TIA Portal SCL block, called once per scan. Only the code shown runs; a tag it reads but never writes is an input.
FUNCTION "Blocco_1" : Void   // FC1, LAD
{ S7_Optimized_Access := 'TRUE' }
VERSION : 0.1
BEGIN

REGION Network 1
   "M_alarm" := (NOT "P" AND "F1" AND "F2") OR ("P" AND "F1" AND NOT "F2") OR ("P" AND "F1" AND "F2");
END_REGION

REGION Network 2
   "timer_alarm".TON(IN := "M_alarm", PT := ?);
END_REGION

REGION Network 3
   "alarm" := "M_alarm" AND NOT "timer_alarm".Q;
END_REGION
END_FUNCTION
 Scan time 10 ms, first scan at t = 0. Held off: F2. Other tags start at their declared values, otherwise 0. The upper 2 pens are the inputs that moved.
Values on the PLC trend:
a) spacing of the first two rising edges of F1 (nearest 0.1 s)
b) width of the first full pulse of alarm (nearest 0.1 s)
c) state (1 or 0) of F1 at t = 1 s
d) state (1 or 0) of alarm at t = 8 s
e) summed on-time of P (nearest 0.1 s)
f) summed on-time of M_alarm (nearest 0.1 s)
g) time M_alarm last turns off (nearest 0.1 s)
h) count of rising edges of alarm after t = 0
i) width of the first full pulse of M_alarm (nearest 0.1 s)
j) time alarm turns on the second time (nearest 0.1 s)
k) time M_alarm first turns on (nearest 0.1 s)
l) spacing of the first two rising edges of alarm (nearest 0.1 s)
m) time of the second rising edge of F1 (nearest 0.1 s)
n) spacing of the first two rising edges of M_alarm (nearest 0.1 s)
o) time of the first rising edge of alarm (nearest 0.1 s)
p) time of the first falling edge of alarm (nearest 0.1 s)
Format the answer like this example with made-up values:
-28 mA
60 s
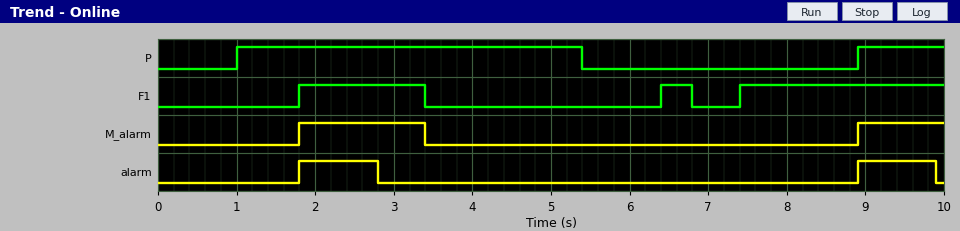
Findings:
4.6 s
1.0 s
0
0
5.5 s
2.7 s
3.4 s
2
1.6 s
8.9 s
1.8 s
7.1 s
6.4 s
7.1 s
1.8 s
2.8 s
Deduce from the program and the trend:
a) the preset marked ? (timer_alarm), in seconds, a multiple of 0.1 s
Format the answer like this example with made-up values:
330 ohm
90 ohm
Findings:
1.0 s
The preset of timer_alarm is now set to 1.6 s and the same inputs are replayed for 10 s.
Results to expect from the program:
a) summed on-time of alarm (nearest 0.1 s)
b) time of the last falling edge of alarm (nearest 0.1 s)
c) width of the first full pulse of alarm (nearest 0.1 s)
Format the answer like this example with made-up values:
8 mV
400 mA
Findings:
2.7 s
3.4 s
1.6 s
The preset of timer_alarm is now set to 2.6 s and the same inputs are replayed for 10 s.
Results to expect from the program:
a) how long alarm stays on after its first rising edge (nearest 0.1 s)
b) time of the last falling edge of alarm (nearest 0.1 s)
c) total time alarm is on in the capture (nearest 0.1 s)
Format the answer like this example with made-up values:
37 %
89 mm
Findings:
1.6 s
3.4 s
2.7 s
